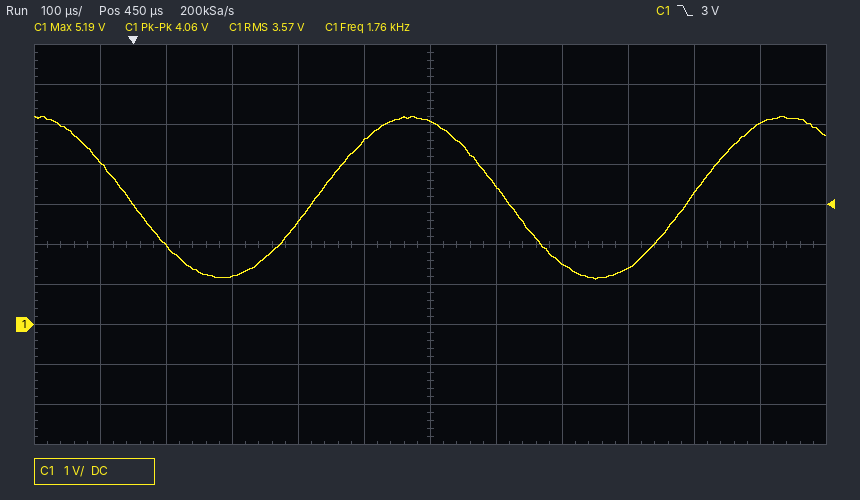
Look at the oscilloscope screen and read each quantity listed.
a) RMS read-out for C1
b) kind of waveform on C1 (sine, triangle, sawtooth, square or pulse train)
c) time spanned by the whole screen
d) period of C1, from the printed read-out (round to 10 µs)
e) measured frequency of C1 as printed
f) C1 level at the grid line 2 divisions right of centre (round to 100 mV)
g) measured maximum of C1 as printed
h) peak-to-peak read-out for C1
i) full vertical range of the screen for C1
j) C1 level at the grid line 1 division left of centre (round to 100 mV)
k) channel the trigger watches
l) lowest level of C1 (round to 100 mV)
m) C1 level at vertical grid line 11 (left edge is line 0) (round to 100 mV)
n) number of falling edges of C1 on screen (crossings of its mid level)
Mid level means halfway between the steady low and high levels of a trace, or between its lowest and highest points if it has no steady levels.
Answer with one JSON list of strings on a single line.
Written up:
["3.57 V", "sine", "1.2 ms", "570 µs", "1.76 kHz", "1.5 V", "5.19 V", "4.06 V", "10 V", "4.6 V", "C1", "1.1 V", "5.0 V", "2"]
